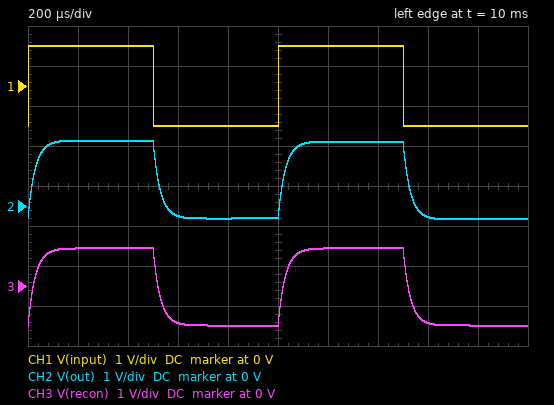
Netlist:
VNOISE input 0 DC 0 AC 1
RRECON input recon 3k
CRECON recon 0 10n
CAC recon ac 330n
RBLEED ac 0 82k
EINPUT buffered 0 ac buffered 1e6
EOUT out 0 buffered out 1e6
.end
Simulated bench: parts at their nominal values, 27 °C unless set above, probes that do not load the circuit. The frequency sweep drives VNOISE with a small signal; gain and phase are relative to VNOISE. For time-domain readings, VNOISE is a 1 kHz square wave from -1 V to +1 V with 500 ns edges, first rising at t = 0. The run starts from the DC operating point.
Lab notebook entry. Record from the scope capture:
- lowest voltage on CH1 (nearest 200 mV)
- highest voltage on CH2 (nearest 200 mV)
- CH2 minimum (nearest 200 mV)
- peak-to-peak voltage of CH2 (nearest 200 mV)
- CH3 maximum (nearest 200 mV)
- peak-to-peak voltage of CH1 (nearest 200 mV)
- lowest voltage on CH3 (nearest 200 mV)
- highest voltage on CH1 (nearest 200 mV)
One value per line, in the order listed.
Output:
-1.0 V
1.6 V
-400 mV
2.0 V
1.0 V
2.0 V
-1.0 V
1.0 V
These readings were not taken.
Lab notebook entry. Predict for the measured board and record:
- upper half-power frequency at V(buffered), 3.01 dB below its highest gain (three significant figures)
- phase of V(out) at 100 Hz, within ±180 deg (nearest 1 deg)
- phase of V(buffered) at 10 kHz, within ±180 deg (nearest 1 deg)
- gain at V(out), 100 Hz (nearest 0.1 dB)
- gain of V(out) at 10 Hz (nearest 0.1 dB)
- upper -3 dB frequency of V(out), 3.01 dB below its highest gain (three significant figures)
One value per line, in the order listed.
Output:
5.51 kHz
2 deg
-61 deg
-0.3 dB
-1.5 dB
5.51 kHz
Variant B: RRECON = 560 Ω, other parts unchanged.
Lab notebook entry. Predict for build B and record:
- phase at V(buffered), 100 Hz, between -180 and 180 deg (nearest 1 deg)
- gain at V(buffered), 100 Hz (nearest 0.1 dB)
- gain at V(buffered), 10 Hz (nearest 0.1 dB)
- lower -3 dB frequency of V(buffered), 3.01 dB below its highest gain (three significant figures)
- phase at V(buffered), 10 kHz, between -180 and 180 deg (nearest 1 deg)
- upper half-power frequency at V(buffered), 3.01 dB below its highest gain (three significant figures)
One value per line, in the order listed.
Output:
3 deg
-0.1 dB
-1.3 dB
5.84 Hz
-19 deg
28.6 kHz
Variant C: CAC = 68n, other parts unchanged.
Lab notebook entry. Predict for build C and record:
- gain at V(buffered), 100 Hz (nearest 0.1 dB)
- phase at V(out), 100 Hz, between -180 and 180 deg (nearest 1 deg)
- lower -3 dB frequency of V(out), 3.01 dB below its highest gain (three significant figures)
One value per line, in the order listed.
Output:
-0.6 dB
14 deg
27.3 Hz
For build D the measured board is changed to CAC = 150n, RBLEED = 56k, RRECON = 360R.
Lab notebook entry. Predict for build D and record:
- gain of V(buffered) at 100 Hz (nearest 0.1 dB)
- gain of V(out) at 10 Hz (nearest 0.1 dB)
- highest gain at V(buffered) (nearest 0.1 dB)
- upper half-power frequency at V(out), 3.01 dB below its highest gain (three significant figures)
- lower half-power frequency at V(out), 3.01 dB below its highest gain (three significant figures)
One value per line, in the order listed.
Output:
-0.2 dB
-6.6 dB
-0.1 dB
44.5 kHz
18.8 Hz
